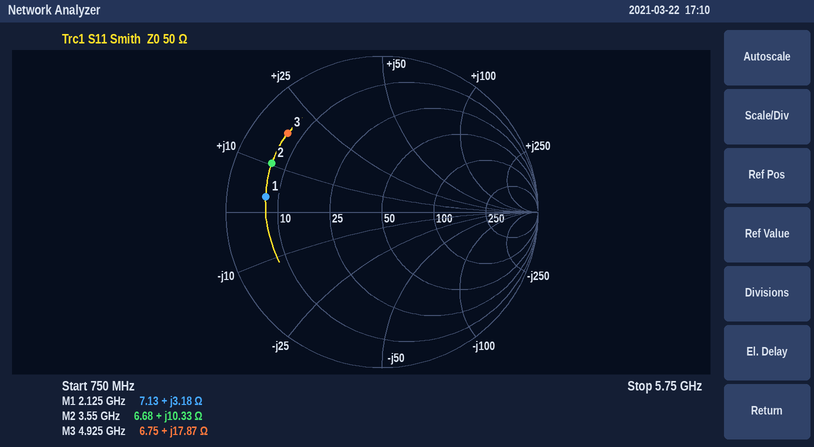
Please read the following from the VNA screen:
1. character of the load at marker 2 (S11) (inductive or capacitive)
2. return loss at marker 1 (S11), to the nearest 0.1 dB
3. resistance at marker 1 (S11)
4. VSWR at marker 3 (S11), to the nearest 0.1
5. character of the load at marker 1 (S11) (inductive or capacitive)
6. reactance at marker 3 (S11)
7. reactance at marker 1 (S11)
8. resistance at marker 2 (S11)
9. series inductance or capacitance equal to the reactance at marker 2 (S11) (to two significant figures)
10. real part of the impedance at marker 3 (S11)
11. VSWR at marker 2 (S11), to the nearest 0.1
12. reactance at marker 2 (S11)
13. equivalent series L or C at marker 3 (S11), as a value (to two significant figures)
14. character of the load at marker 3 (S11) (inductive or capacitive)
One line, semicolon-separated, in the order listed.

inductive; 2.5 dB; 7.13 Ω; 8.4; inductive; +17.87 Ω; +3.18 Ω; 6.68 Ω; 460 pH; 6.75 Ω; 7.8; +10.33 Ω; 580 pH; inductive
